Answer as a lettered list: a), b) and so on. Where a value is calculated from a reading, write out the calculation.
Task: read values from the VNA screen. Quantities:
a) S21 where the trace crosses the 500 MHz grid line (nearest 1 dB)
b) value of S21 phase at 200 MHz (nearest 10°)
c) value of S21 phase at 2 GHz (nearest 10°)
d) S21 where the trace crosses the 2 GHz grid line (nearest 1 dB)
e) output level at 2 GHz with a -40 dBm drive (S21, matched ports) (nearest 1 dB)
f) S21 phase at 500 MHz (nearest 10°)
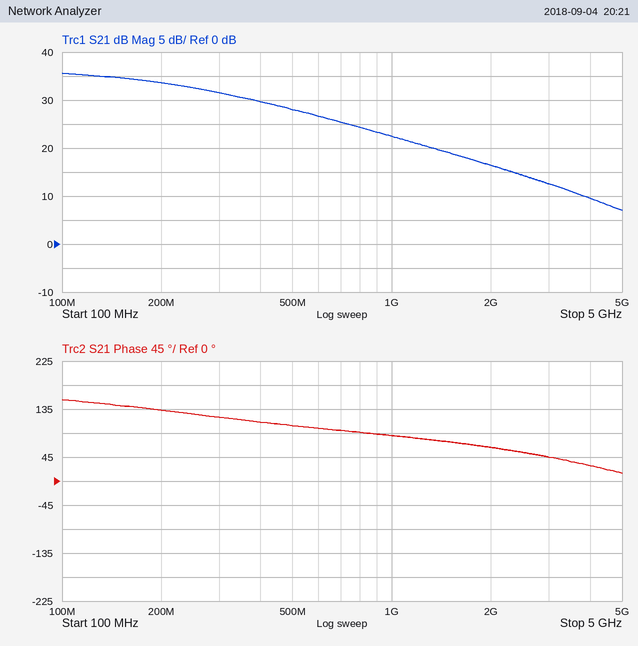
a) 28 dB
b) 130°
c) 60°
d) 16 dB
e) -40 dBm + (16 dB) = -24 dBm
f) 100°
